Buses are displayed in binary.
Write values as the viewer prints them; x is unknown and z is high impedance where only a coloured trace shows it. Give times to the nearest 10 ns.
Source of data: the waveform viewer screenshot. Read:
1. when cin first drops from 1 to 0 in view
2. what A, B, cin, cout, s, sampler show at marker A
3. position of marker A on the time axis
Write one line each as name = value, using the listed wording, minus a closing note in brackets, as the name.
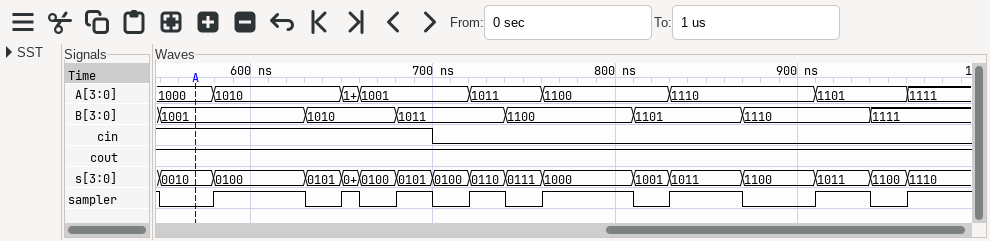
when cin first drops from 1 to 0 in view = 700 ns
what A, B, cin, cout, s, sampler show at marker A = A=1000, B=1001, cin=1, cout=1, s=0010, sampler=0
position of marker A on the time axis = 570 ns
